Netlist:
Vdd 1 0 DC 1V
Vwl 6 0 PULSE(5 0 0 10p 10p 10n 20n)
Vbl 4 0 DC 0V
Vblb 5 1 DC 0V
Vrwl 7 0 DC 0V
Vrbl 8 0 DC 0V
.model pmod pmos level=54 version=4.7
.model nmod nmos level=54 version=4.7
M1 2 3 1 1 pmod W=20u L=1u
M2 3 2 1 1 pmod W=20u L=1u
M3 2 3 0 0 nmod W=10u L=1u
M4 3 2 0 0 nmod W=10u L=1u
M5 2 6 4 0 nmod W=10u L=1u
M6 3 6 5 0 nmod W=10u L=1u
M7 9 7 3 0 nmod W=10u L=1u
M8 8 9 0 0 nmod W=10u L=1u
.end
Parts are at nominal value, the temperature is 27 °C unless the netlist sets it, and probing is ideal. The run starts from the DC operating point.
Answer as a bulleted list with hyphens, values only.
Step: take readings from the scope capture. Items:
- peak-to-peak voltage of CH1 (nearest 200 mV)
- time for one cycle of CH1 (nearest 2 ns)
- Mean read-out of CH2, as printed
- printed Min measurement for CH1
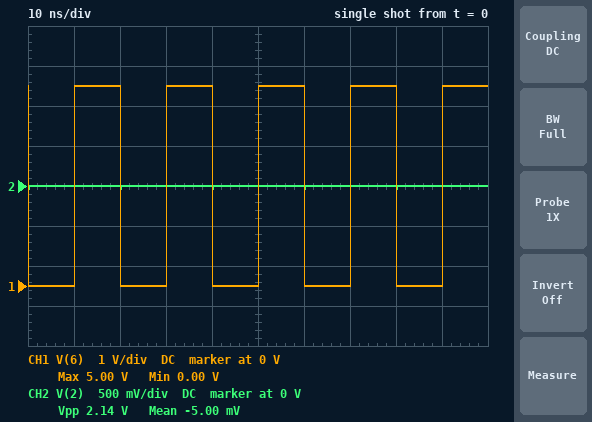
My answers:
- 5.0 V
- 20 ns
- -5.00 mV
- 0.00 V
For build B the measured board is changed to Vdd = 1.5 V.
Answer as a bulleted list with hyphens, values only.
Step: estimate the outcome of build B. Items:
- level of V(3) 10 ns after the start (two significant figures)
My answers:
- 1.5 V
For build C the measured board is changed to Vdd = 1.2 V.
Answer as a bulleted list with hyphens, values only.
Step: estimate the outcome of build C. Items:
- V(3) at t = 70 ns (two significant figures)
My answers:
- 1.2 V
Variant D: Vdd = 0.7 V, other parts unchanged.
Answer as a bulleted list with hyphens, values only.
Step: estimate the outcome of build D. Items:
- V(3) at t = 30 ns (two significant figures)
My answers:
- 700 mV
